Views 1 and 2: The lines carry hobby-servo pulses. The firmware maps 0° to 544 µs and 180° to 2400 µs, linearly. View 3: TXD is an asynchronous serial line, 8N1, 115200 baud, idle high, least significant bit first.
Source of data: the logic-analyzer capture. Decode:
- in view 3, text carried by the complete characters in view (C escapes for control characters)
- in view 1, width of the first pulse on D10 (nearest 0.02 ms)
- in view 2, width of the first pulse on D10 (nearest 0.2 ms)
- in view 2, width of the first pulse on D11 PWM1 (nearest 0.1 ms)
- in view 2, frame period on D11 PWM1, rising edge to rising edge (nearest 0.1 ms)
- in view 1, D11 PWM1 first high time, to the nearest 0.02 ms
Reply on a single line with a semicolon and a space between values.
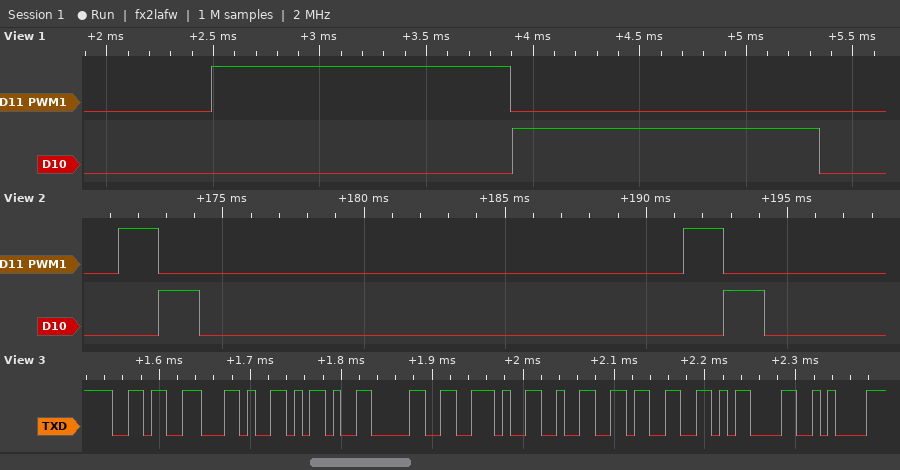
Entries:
"6,-0.23\r\n"; 1.44 ms; 1.4 ms; 1.4 ms; 20.0 ms; 1.40 ms
